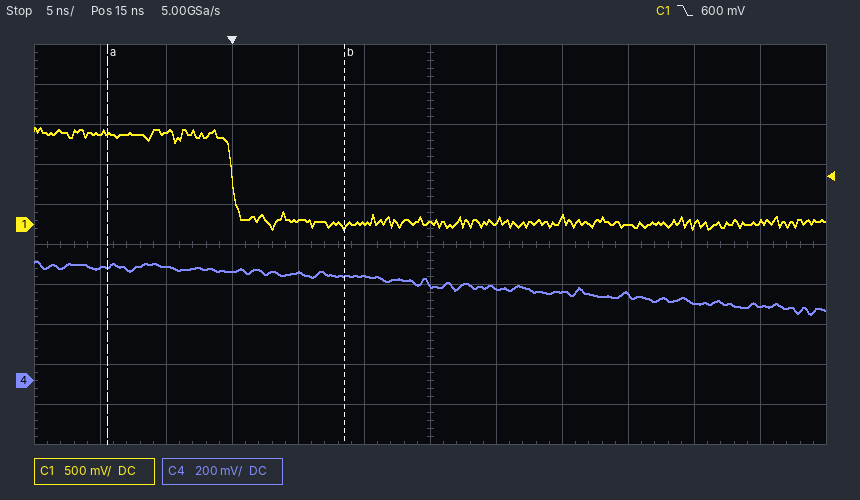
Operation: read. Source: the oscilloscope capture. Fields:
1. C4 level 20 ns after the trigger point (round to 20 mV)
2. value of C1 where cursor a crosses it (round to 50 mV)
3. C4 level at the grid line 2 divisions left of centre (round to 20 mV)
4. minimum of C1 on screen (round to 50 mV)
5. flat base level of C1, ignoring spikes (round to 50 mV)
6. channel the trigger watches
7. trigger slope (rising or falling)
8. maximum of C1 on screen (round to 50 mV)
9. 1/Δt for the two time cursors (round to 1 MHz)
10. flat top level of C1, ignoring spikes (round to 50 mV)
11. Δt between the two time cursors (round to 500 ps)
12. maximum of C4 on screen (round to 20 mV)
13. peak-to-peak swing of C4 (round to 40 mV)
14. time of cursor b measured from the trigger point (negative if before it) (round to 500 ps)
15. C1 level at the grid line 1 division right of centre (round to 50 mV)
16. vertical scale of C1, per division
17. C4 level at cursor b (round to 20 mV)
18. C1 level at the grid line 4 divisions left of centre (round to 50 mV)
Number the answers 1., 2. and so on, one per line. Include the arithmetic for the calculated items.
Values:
1. 460 mV
2. 1.15 V
3. 540 mV
4. -50 mV
5. 0 mV
6. C1
7. falling
8. 1.20 V
9. 1 / 18.0 ns ≈ 56 MHz
10. 1.15 V
11. 18.0 ns
12. 600 mV
13. 280 mV
14. +8.5 ns
15. 50 mV
16. 500 mV
17. 520 mV
18. 1.15 V
